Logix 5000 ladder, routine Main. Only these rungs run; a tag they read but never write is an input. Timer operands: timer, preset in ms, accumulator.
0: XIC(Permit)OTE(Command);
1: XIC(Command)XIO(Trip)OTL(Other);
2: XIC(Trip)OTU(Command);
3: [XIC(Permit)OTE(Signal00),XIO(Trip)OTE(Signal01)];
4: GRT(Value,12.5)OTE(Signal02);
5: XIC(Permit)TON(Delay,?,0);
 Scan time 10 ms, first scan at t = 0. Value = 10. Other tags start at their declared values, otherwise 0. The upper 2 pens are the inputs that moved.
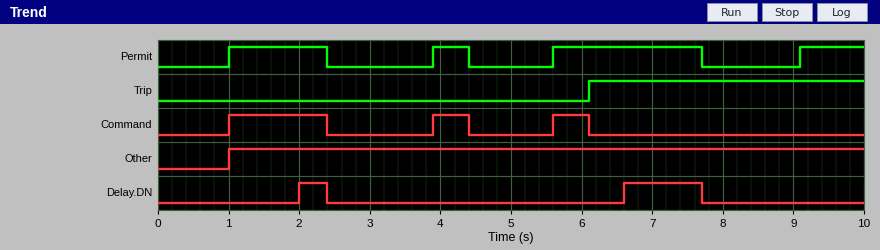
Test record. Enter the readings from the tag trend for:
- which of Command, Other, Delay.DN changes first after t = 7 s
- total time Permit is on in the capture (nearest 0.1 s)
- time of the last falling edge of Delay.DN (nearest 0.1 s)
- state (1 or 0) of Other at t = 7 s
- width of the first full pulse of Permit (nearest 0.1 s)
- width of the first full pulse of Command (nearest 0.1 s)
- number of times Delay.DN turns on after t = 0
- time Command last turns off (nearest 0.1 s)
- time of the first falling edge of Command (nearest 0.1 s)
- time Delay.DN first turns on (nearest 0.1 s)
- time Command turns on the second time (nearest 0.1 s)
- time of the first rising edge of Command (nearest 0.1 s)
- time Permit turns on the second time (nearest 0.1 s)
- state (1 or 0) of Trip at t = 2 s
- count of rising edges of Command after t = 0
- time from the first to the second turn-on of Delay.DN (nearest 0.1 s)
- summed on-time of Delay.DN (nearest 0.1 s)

Delay.DN
4.9 s
7.7 s
1
1.4 s
1.4 s
2
6.1 s
2.4 s
2.0 s
3.9 s
1.0 s
3.9 s
0
3
4.6 s
1.5 s
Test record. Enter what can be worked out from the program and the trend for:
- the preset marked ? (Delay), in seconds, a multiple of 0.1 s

1.0 s
